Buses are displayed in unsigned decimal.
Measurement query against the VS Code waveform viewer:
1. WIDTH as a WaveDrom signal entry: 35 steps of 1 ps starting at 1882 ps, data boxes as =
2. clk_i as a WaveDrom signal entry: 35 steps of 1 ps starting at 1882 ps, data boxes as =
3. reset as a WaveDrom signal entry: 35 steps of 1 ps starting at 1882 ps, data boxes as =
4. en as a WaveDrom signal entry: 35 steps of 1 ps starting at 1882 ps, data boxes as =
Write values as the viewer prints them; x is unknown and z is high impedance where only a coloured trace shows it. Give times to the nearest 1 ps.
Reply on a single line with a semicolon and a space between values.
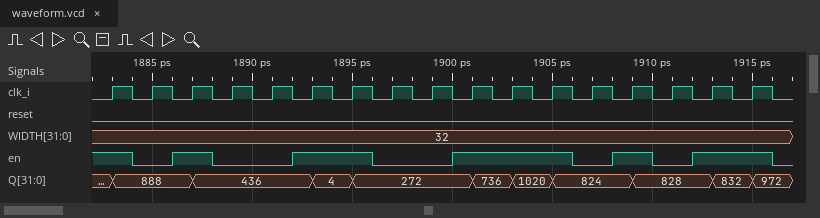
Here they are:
{name: 'WIDTH', wave: '=..................................', data: '32'}; {name: 'clk_i', wave: '01010101010101010101010101010101010'}; {name: 'reset', wave: '0..................................'}; {name: 'en', wave: '1.0.1.0...1...0...1.....0.1.0.1...0'}
